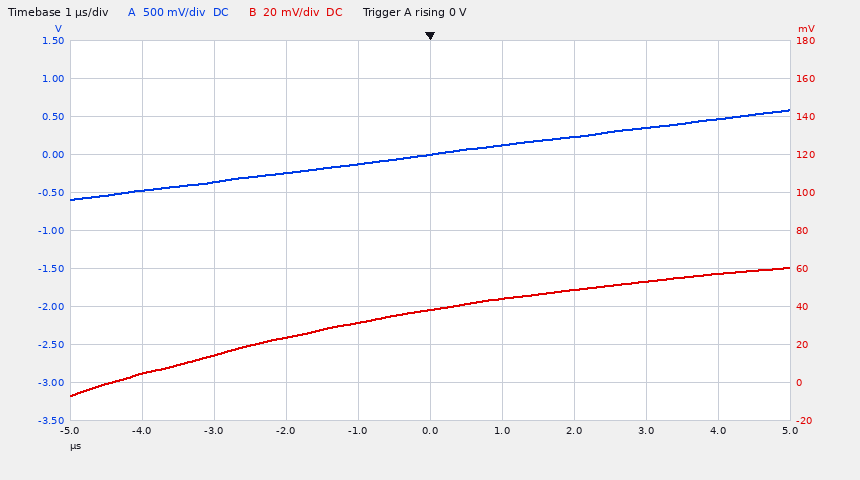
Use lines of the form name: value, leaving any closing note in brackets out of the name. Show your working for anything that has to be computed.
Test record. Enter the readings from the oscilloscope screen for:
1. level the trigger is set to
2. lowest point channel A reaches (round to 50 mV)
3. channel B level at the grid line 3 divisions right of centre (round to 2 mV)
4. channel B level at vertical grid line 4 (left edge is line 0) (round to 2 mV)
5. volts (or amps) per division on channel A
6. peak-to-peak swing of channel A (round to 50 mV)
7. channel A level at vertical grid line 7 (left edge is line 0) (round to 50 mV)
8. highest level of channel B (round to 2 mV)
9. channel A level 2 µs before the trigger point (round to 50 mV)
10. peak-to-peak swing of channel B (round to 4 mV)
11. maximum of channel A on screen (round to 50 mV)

level the trigger is set to: 0 V
lowest point channel A reaches: -600 mV
channel B level at the grid line 3 divisions right of centre: 54 mV
channel B level at vertical grid line 4 (left edge is line 0): 32 mV
volts (or amps) per division on channel A: 500 mV
peak-to-peak swing of channel A: 600 mV − (-600 mV) = 1.20 V
channel A level at vertical grid line 7 (left edge is line 0): 250 mV
highest level of channel B: 60 mV
channel A level 2 µs before the trigger point: -250 mV
peak-to-peak swing of channel B: 68 mV
maximum of channel A on screen: 600 mV
